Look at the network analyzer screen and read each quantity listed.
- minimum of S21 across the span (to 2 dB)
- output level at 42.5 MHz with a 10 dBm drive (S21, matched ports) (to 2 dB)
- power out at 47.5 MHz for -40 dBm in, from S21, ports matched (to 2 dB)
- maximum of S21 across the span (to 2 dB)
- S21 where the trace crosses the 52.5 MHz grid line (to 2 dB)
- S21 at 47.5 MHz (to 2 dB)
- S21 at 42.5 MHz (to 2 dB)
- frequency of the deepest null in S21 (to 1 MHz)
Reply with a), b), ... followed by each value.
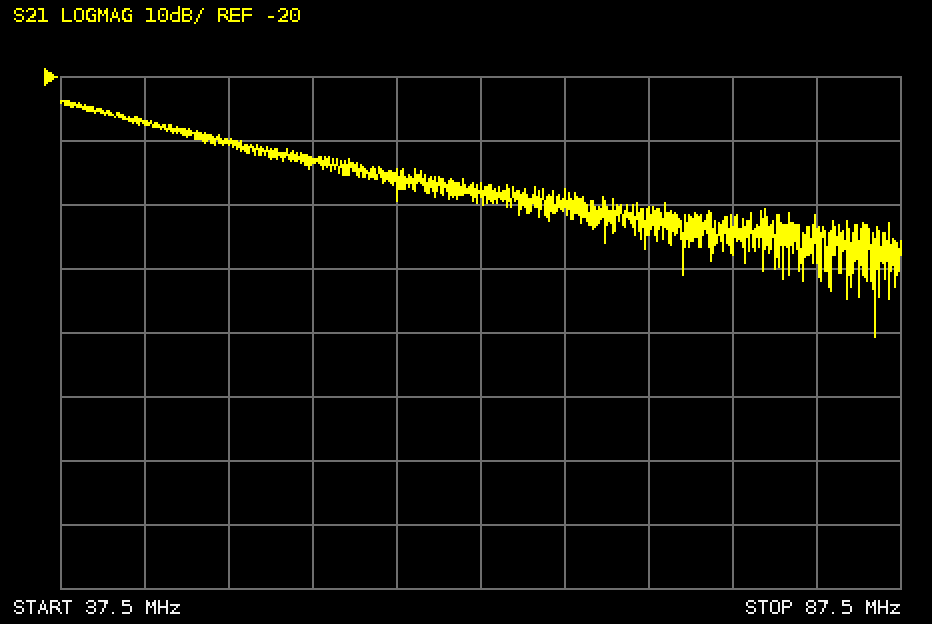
a) -60 dB
b) -18 dBm
c) -70 dBm
d) -24 dB
e) -34 dB
f) -30 dB
g) -28 dB
h) 86 MHz
